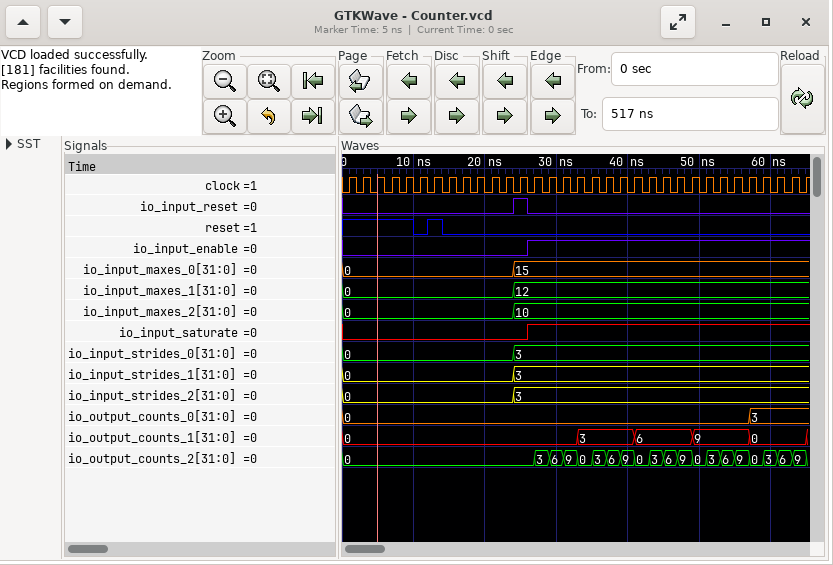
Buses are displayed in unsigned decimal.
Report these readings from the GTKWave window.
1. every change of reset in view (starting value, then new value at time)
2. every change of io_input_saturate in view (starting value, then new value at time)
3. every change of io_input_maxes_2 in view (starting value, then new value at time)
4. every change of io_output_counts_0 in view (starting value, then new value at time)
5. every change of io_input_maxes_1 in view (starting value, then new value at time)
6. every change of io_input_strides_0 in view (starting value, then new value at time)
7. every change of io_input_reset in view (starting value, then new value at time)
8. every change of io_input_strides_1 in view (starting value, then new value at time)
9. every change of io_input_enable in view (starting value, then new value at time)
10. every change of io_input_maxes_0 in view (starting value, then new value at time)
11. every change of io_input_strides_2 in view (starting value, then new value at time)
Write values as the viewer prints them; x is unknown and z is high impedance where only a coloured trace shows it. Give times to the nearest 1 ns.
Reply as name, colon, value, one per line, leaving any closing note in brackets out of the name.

every change of reset in view: 1, 0 at 10 ns, 1 at 12 ns, 0 at 14 ns
every change of io_input_saturate in view: 0, 1 at 26 ns
every change of io_input_maxes_2 in view: 0, 10 at 24 ns
every change of io_output_counts_0 in view: 0, 3 at 57 ns
every change of io_input_maxes_1 in view: 0, 12 at 24 ns
every change of io_input_strides_0 in view: 0, 3 at 24 ns
every change of io_input_reset in view: 0, 1 at 24 ns, 0 at 26 ns
every change of io_input_strides_1 in view: 0, 3 at 24 ns
every change of io_input_enable in view: 0, 1 at 26 ns
every change of io_input_maxes_0 in view: 0, 15 at 24 ns
every change of io_input_strides_2 in view: 0, 3 at 24 ns
